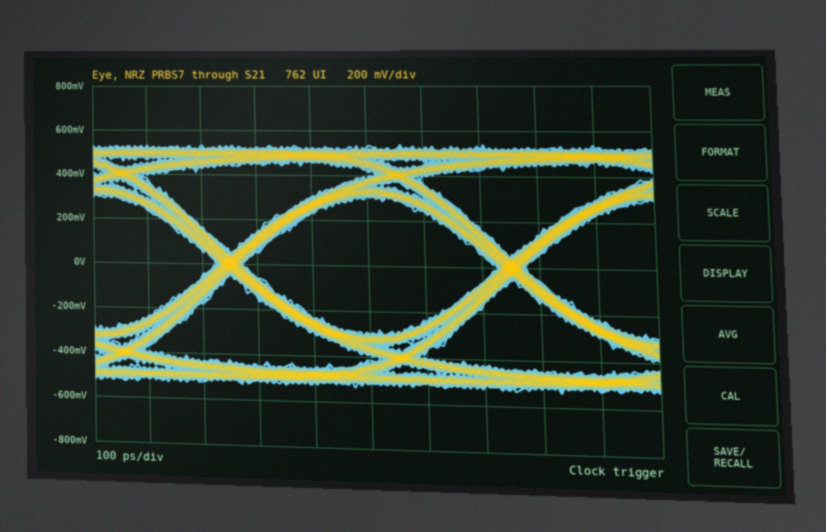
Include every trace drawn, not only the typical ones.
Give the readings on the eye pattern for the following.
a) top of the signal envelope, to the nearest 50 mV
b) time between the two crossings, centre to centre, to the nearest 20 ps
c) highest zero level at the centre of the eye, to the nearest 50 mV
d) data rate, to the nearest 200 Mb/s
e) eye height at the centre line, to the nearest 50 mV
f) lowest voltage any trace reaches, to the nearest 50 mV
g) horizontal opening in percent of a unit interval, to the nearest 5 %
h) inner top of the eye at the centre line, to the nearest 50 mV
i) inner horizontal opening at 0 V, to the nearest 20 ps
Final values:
550 mV
500 ps
-300 mV
2.0 Gb/s
600 mV
-550 mV
90 %
300 mV
460 ps
